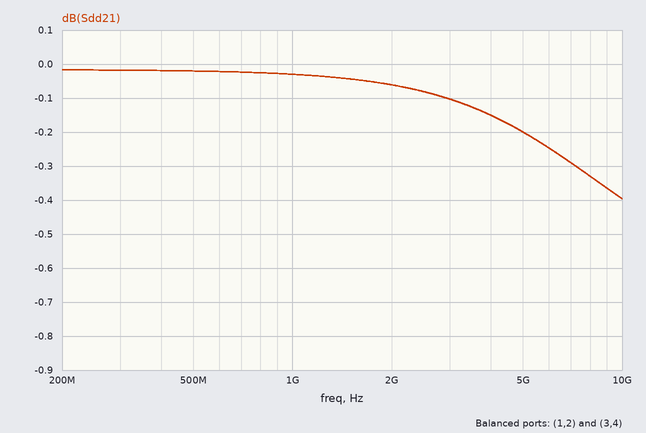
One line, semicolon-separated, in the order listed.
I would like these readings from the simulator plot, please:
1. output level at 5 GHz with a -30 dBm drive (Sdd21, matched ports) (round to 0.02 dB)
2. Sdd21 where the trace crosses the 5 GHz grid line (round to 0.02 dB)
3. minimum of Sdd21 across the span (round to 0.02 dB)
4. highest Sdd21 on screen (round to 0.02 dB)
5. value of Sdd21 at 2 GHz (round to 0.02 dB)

-30.20 dBm; -0.20 dB; -0.40 dB; -0.02 dB; -0.06 dB
